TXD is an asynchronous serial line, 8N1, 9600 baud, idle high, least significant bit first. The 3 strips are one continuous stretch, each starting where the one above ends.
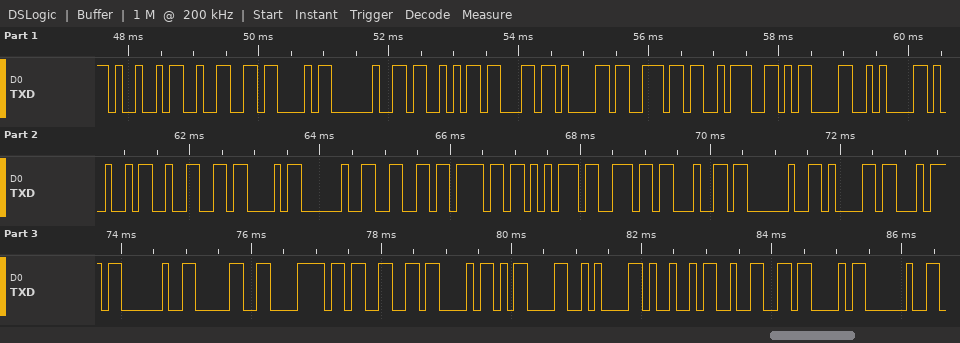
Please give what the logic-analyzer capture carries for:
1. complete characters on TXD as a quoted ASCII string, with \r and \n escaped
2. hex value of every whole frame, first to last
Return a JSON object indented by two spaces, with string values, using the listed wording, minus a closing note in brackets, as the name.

{
  "complete characters on TXD as a quoted ASCII string, with \\r and \\n escaped": "\"I2C Scan:\\r\\nI2C found at 0x3C\\r\\nI2C \"",
  "hex value of every whole frame, first to last": "49 32 43 20 53 63 61 6E 3A 0D 0A 49 32 43 20 66 6F 75 6E 64 20 61 74 20 30 78 33 43 0D 0A 49 32 43 20"
}
